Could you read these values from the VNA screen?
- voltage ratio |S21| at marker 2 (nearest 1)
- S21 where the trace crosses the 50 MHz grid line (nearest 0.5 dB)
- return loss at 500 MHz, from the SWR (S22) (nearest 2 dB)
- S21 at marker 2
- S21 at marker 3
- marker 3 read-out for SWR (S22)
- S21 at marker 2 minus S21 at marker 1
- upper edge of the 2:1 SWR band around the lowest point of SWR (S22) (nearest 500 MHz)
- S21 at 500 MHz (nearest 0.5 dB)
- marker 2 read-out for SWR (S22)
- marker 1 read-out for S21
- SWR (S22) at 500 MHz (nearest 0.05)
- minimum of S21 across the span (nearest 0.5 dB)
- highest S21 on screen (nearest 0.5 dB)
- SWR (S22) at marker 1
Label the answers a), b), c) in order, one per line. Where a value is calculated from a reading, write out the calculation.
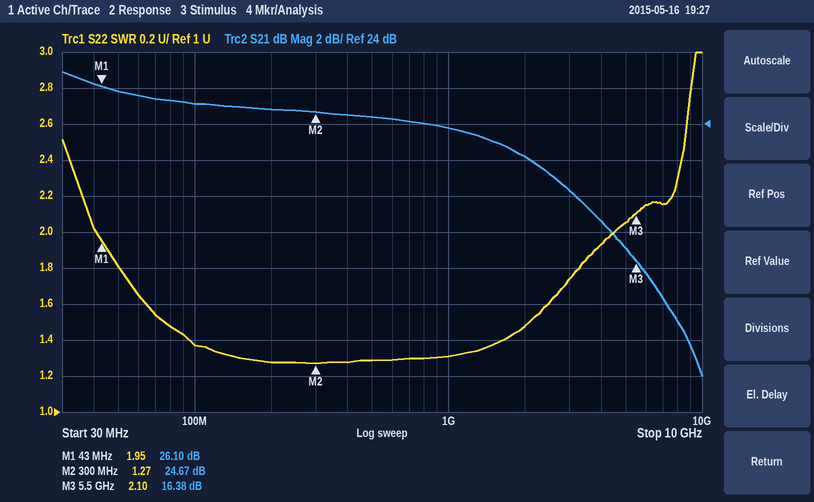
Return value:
a) 10^(24.67/20) ≈ 17
b) 26.0 dB
c) −20 log10((1.3 − 1)/(1.3 + 1)) ≈ 18 dB
d) 24.67 dB
e) 16.38 dB
f) 2.10
g) 24.67 − (26.1) = -1.43 dB
h) 4.5 GHz
i) 24.5 dB
j) 1.27
k) 26.10 dB
l) 1.30
m) 10.0 dB
n) 27.0 dB
o) 1.95
